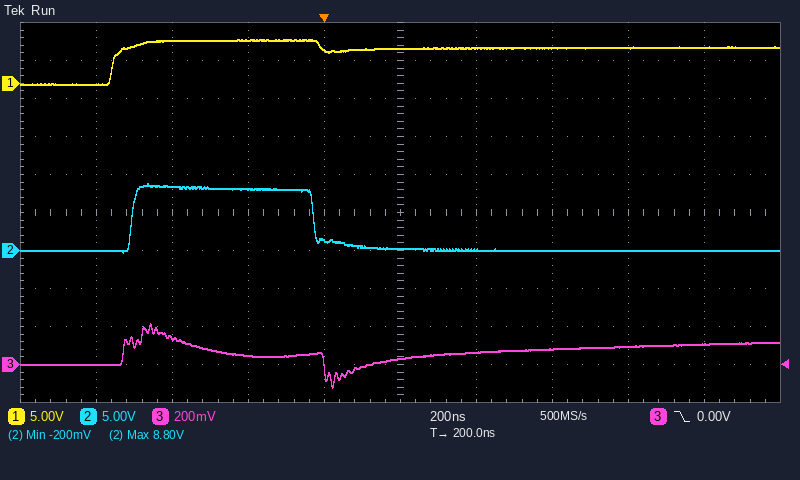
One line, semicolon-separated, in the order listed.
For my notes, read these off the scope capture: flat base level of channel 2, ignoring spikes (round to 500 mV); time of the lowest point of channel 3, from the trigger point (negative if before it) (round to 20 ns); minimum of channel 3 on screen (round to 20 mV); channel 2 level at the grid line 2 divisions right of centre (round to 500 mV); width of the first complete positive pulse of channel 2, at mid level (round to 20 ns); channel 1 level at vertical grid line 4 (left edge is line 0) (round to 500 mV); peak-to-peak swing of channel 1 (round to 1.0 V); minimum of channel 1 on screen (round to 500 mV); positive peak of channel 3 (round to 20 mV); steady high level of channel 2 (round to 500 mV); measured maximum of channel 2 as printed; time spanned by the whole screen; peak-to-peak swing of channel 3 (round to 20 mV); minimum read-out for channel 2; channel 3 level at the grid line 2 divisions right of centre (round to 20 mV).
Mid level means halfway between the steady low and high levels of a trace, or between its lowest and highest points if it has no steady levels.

0.0 V; +20 ns; -120 mV; 0.0 V; 480 ns; 4.5 V; 6.0 V; 0.0 V; 220 mV; 8.0 V; 8.80 V; 2 µs; 340 mV; -200 mV; 80 mV
